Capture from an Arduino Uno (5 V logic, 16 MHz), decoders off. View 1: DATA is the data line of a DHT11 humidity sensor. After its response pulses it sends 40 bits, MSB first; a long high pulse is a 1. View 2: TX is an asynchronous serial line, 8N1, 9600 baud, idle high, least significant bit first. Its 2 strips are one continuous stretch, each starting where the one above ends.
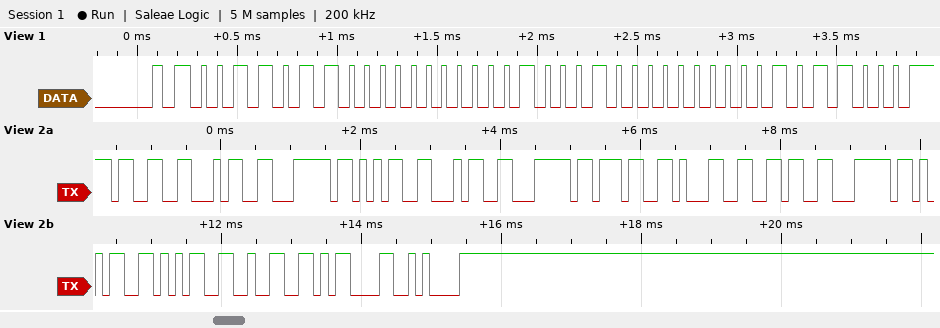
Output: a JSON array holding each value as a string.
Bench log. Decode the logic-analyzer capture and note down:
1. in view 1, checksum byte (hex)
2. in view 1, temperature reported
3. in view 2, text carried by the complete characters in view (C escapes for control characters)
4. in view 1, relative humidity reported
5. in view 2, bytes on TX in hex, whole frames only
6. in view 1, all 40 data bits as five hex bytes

["0x58", "34.0 °C", "\"34|54|716|552\\r\\n\"", "54 %", "33 34 7C 35 34 7C 37 31 36 7C 35 35 32 0D 0A", "36 00 22 00 58"]
